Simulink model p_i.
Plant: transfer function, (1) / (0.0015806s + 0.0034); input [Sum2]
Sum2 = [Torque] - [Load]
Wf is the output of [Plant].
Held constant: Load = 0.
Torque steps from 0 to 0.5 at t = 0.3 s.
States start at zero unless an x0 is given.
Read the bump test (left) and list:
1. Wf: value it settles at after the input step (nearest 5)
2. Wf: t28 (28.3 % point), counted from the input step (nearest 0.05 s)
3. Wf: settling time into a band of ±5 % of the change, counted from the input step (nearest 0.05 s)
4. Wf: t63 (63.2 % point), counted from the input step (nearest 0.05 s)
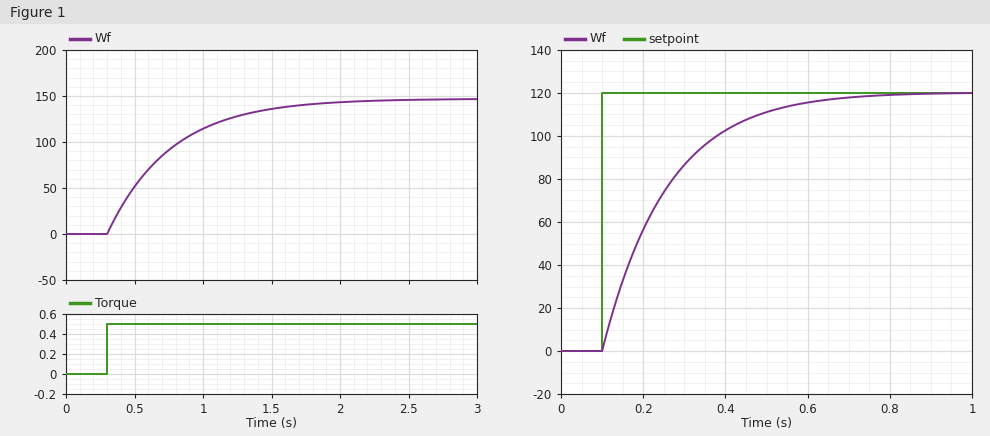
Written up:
145
0.15 s
1.40 s
0.45 s
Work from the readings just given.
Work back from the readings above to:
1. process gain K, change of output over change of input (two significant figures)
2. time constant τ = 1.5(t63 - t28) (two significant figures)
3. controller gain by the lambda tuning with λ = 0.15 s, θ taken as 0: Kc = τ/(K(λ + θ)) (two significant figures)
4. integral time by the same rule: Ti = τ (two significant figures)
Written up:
290
0.45 s
0.010
0.45 s
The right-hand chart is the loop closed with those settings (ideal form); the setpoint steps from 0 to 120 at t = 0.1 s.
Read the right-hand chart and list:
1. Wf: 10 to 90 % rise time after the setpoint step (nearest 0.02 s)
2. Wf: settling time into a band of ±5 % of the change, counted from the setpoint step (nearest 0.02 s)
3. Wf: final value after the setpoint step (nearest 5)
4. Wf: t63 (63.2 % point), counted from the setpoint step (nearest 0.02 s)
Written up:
0.34 s
0.46 s
120
0.16 s
